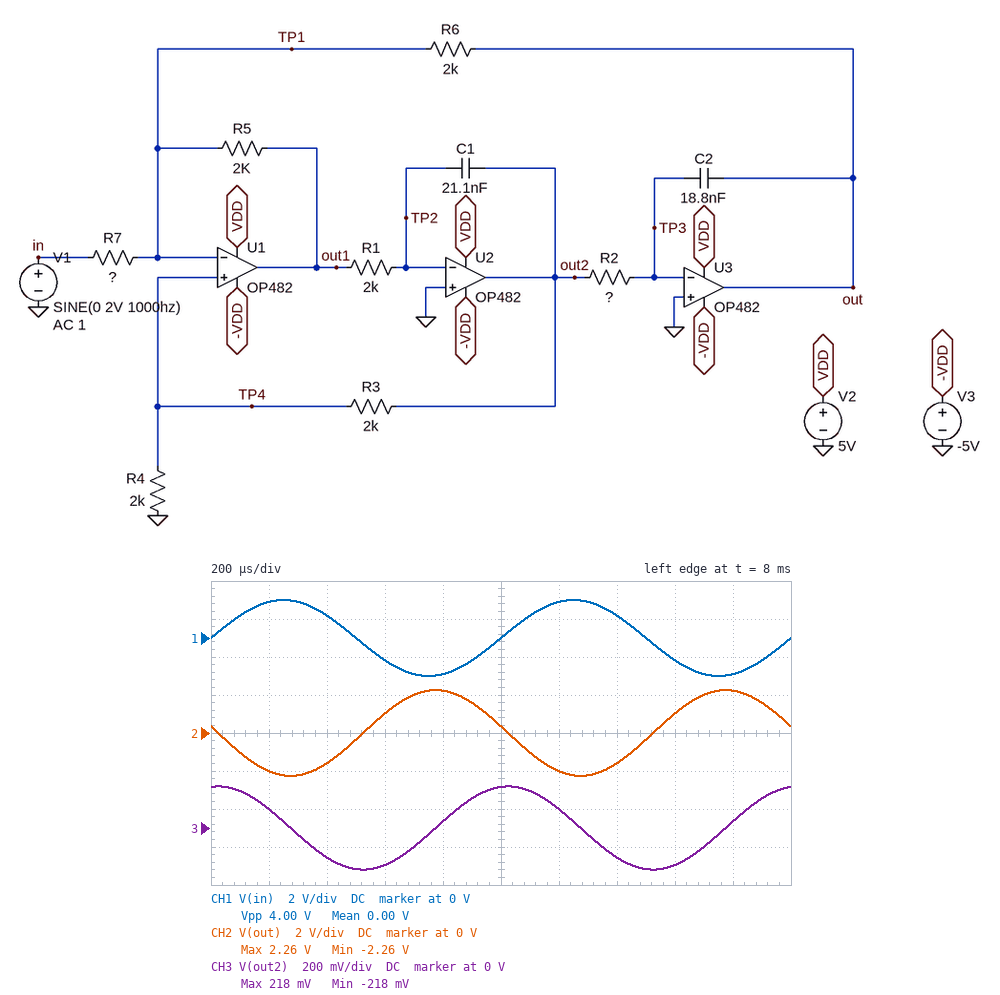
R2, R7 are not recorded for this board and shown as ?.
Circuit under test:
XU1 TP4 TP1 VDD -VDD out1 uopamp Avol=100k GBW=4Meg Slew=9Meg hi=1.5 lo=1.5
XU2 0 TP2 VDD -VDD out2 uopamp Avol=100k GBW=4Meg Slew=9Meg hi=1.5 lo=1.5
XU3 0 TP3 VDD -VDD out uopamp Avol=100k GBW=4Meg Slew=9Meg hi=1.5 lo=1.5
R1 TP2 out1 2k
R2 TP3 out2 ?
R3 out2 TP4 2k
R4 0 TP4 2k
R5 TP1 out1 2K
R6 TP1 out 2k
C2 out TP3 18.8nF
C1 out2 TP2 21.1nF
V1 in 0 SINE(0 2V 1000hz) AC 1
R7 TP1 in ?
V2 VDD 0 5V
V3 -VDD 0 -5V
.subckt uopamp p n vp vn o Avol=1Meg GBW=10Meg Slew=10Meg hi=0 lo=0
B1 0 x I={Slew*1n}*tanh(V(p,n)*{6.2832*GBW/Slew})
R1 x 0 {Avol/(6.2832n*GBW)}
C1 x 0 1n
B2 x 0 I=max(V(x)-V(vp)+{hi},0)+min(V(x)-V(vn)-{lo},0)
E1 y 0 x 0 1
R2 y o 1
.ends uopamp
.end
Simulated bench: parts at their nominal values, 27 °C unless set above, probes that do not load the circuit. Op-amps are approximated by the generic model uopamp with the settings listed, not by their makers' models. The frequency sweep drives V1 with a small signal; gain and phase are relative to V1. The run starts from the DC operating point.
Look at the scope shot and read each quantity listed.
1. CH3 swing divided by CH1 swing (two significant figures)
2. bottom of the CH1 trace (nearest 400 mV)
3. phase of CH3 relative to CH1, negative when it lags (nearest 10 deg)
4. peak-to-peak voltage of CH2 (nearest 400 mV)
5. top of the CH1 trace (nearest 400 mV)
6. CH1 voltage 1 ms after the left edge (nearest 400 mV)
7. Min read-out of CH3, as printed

0.11
-2.0 V
80 deg
4.4 V
2.0 V
0 V
-218 mV
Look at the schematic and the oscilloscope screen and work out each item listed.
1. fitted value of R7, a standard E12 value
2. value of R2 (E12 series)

1.8 kΩ
820 Ω
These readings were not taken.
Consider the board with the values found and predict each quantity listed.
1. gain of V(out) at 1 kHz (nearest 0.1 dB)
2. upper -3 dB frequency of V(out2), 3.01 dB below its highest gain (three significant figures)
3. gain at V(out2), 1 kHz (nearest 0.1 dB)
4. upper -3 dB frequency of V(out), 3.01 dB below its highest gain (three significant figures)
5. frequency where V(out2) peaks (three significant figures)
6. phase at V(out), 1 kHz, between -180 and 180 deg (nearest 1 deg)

1.0 dB
9.82 kHz
-19.2 dB
7.36 kHz
6.25 kHz
171 deg
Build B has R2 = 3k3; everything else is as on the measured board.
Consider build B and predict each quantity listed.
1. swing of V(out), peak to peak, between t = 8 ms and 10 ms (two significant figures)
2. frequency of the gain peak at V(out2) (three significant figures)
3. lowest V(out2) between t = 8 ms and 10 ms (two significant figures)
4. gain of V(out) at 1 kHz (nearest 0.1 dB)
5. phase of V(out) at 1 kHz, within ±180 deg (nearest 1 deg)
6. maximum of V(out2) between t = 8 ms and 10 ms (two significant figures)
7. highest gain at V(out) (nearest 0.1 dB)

4.1 V
3.12 kHz
-800 mV
0.2 dB
146 deg
800 mV
0.9 dB
